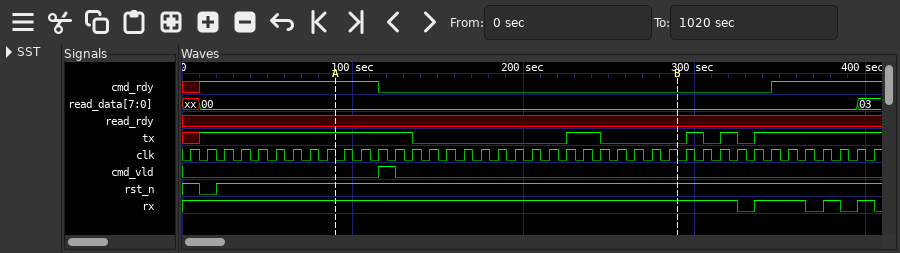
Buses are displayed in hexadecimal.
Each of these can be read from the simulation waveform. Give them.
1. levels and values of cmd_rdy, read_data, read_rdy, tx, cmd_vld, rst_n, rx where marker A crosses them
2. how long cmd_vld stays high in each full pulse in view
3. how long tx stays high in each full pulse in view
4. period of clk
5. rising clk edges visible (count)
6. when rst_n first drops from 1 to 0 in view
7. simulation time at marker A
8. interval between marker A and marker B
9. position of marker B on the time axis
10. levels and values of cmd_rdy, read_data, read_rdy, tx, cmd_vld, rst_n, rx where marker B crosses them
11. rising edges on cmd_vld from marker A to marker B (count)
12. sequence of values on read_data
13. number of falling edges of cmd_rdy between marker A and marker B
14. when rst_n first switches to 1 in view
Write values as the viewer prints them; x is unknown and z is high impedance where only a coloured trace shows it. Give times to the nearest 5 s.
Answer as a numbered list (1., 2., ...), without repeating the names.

1. cmd_rdy=1, read_data=00, read_rdy=x, tx=1, cmd_vld=0, rst_n=1, rx=1
2. 10 s
3. 20 s, 10 s, 10 s
4. 10 s
5. 41
6. 10 s
7. 90 s
8. 200 s
9. 290 s
10. cmd_rdy=0, read_data=00, read_rdy=x, tx=0, cmd_vld=0, rst_n=1, rx=1
11. 1
12. xx, 00, 03
13. 1
14. 20 s
